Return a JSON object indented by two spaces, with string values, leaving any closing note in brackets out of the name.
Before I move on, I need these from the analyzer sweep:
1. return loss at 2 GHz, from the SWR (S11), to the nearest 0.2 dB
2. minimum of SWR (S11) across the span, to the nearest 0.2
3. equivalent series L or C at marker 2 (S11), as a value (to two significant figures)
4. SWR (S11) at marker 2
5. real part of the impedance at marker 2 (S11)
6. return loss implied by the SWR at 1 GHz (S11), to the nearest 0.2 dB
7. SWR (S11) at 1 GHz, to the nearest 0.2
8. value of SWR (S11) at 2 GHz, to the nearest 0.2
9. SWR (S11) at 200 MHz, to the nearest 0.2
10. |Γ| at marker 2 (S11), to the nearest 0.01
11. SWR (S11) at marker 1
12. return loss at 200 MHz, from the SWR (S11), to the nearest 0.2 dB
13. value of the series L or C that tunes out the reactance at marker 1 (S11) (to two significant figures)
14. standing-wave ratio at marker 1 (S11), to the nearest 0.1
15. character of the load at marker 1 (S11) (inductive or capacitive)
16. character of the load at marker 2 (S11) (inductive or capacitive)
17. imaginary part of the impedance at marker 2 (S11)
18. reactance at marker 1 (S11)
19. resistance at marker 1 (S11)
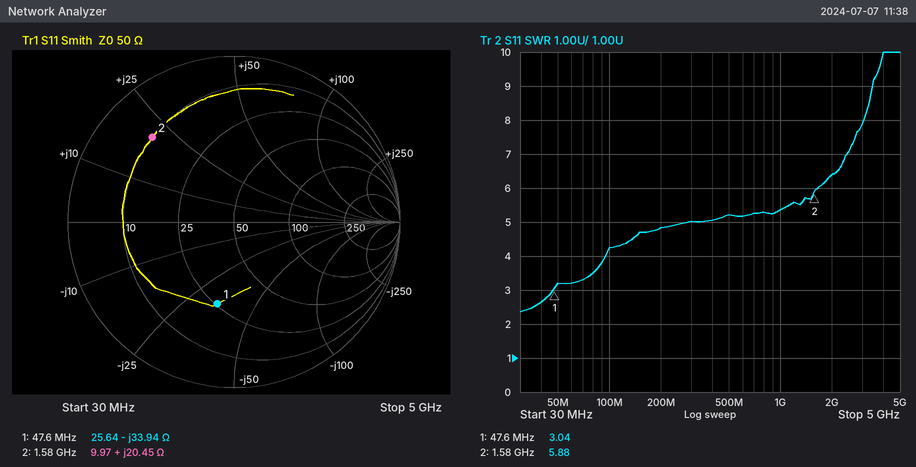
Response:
{
  "return loss at 2 GHz, from the SWR (S11), to the nearest 0.2 dB": "2.8 dB",
  "minimum of SWR (S11) across the span, to the nearest 0.2": "2.4",
  "equivalent series L or C at marker 2 (S11), as a value": "2.1 nH",
  "SWR (S11) at marker 2": "5.88",
  "real part of the impedance at marker 2": "9.97 Ω",
  "return loss implied by the SWR at 1 GHz (S11), to the nearest 0.2 dB": "3.2 dB",
  "SWR (S11) at 1 GHz, to the nearest 0.2": "5.4",
  "value of SWR (S11) at 2 GHz, to the nearest 0.2": "6.4",
  "SWR (S11) at 200 MHz, to the nearest 0.2": "4.8",
  "|Γ| at marker 2 (S11), to the nearest 0.01": "0.71",
  "SWR (S11) at marker 1": "3.04",
  "return loss at 200 MHz, from the SWR (S11), to the nearest 0.2 dB": "3.6 dB",
  "value of the series L or C that tunes out the reactance at marker 1 (S11)": "110 nH",
  "standing-wave ratio at marker 1 (S11), to the nearest 0.1": "3.0",
  "character of the load at marker 1 (S11)": "capacitive",
  "character of the load at marker 2 (S11)": "inductive",
  "imaginary part of the impedance at marker 2": "+20.45 Ω",
  "reactance at marker 1": "-33.94 Ω",
  "resistance at marker 1": "25.64 Ω"
}
